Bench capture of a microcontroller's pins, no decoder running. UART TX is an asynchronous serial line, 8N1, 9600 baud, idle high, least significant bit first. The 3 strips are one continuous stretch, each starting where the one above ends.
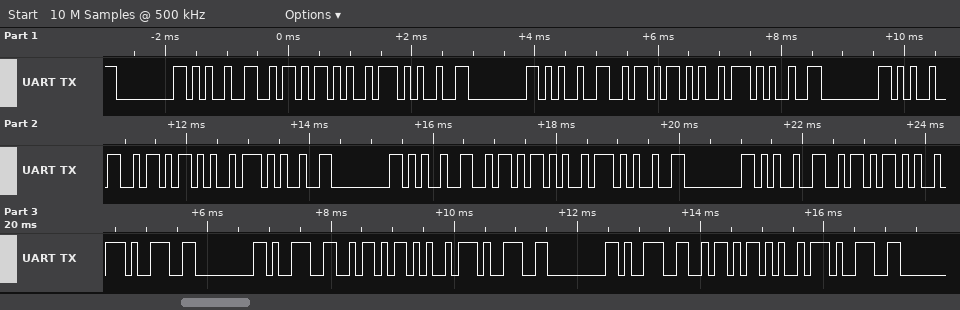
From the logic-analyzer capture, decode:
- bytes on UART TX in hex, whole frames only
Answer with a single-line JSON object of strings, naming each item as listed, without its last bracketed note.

{"bytes on UART TX in hex, whole frames only": "00 25 5A A5 25 00 25 5A A5 25 00 25 5A A5 25 00 25 5A A5 25 00 25 5A A5 39 00 39 5A A5 39 00 39 5A A5 39"}
